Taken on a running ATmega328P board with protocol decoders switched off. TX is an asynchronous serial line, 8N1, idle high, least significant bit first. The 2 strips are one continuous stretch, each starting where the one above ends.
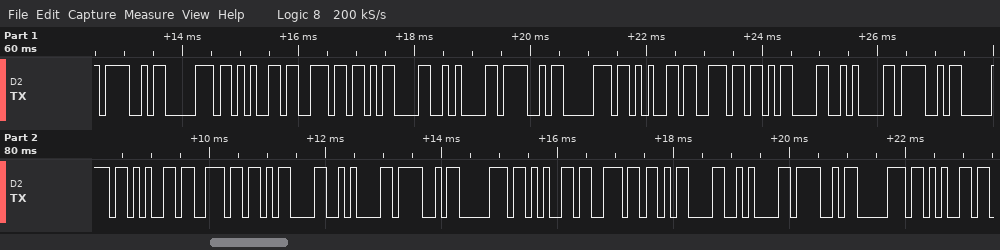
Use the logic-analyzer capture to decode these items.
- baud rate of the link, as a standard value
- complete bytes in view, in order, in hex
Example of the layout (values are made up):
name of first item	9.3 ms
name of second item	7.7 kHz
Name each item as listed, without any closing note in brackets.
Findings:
baud rate of the link, as a standard value	9600 baud
complete bytes in view, in order, in hex	4F 70 65 6E 0D 0A 4F 70 65 6E 0D 0A 4F 70 65 6E 0D 0A 4F 70 65 6E 0D 0A 4F 70 65
